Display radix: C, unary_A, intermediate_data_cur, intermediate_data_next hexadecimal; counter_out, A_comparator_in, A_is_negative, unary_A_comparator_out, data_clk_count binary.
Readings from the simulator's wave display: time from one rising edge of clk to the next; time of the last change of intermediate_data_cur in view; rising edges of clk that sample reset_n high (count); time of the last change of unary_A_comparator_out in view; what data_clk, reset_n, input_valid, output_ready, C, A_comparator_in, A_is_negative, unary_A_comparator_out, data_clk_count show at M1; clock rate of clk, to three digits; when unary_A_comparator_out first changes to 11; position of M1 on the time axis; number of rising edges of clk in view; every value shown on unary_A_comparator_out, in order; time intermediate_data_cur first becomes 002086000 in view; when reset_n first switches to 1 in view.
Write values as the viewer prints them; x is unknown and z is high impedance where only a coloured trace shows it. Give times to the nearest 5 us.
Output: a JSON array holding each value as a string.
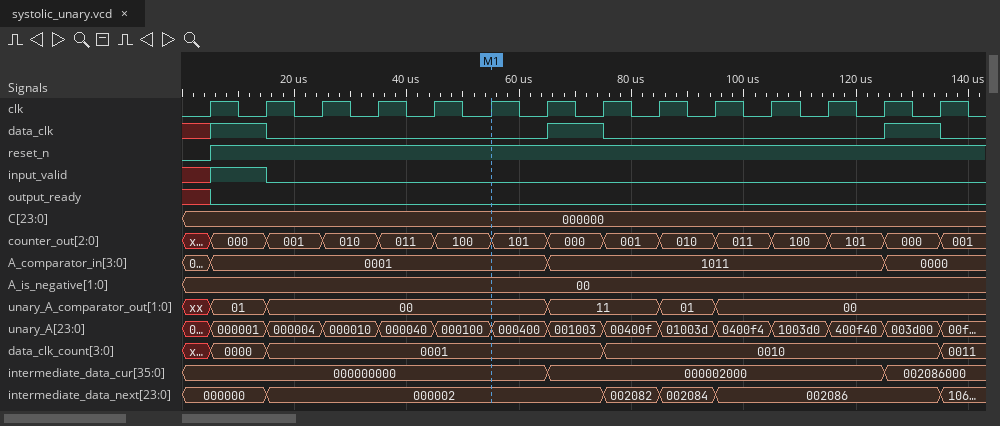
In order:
["10 us", "125 us", "13", "95 us", "data_clk=0, reset_n=1, input_valid=0, output_ready=0, C=000000, A_comparator_in=0001, A_is_negative=00, unary_A_comparator_out=00, data_clk_count=0001", "100 kHz", "65 us", "55 us", "14", "xx, 01, 00, 11, 01, 00", "125 us", "5 us"]
